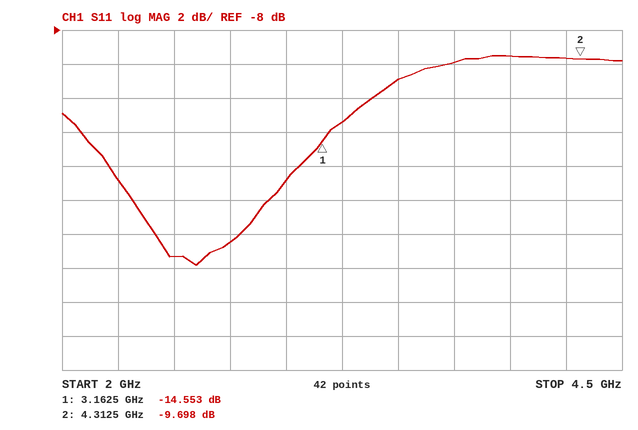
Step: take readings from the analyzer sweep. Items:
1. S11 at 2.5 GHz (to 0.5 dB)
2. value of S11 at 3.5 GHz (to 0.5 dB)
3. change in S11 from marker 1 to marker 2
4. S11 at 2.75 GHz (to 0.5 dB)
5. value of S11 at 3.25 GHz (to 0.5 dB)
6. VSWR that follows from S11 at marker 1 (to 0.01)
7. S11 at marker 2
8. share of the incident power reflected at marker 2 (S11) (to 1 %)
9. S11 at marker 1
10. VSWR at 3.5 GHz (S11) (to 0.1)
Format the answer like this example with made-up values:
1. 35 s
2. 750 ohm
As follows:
1. -21.5 dB
2. -11.0 dB
3. 4.855 dB
4. -20.5 dB
5. -13.5 dB
6. 1.46
7. -9.698 dB
8. 11 %
9. -14.553 dB
10. 1.8
